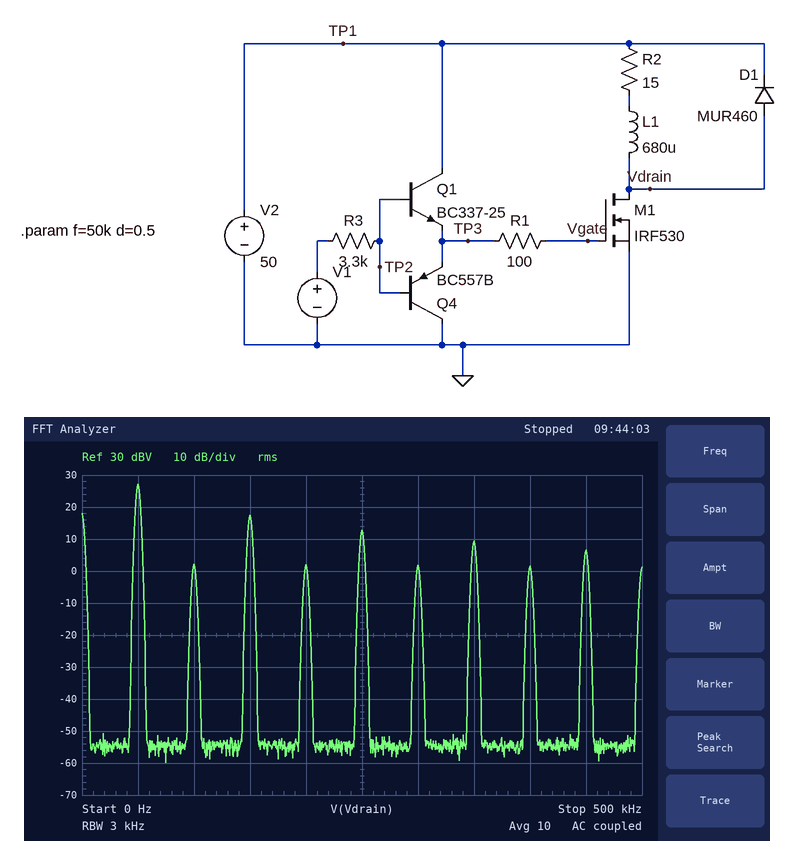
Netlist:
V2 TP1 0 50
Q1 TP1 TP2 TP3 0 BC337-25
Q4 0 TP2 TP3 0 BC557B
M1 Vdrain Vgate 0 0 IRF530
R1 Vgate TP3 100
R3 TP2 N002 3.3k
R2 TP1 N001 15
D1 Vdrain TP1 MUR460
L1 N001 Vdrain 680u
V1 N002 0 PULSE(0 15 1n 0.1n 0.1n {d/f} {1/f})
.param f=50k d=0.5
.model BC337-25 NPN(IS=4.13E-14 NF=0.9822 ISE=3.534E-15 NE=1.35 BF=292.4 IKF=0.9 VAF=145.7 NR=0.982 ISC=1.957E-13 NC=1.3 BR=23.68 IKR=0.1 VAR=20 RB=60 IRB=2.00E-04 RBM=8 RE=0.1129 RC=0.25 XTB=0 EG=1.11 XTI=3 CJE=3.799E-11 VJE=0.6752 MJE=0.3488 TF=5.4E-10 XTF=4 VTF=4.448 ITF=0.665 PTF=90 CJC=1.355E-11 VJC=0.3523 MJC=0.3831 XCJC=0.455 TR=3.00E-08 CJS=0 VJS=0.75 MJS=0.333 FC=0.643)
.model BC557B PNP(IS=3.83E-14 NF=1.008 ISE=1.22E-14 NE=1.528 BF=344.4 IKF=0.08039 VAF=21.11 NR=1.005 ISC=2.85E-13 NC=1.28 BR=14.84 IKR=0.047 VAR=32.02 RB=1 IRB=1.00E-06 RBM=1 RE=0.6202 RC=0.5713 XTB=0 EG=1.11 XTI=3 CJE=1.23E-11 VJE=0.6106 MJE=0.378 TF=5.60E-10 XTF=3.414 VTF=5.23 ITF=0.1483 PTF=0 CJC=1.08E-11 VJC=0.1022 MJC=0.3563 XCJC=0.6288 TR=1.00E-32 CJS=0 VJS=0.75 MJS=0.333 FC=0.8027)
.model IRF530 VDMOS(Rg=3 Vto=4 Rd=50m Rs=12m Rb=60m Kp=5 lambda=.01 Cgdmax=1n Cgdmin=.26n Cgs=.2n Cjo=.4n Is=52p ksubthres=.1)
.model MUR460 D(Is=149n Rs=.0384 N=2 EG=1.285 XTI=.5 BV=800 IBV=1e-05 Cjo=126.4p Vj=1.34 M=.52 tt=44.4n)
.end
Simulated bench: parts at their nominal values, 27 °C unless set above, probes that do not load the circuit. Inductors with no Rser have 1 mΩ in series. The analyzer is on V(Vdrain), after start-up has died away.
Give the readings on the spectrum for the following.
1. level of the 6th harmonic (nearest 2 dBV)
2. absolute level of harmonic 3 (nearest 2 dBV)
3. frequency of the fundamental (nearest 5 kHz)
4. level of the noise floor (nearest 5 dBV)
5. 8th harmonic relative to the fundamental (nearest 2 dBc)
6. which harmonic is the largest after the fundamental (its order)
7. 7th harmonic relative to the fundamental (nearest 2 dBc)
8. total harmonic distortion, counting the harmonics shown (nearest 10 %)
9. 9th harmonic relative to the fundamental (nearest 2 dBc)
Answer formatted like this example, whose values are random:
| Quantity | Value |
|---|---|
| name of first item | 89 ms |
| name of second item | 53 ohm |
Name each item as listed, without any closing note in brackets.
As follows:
| Quantity | Value |
|---|---|
| level of the 6th harmonic | 2 dBV |
| absolute level of harmonic 3 | 18 dBV |
| frequency of the fundamental | 50 kHz |
| level of the noise floor | -55 dBV |
| 8th harmonic relative to the fundamental | -26 dBc |
| which harmonic is the largest after the fundamental | 3 |
| 7th harmonic relative to the fundamental | -18 dBc |
| total harmonic distortion, counting the harmonics shown | 40 % |
| 9th harmonic relative to the fundamental | -20 dBc |
